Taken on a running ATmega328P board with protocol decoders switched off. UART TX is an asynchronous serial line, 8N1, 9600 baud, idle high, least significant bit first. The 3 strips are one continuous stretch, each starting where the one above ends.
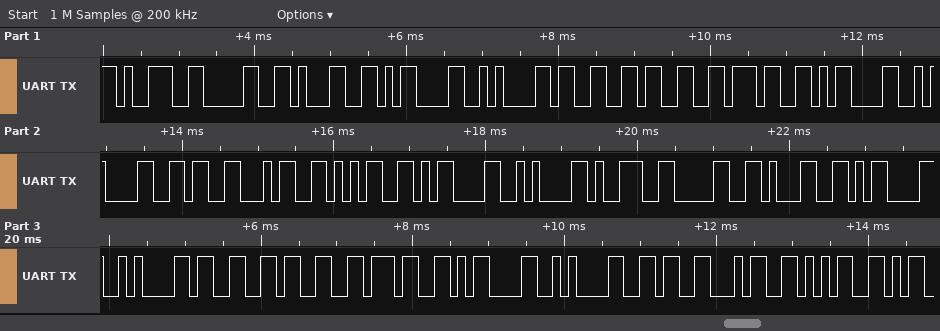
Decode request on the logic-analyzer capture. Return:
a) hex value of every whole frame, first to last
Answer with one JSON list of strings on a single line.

["39 30 31 0D 0A 33 33 37 0D 0A 36 34 35 0D 0A 39 30 31 0D 0A 33 33 37 0D 0A 36 34 35"]
